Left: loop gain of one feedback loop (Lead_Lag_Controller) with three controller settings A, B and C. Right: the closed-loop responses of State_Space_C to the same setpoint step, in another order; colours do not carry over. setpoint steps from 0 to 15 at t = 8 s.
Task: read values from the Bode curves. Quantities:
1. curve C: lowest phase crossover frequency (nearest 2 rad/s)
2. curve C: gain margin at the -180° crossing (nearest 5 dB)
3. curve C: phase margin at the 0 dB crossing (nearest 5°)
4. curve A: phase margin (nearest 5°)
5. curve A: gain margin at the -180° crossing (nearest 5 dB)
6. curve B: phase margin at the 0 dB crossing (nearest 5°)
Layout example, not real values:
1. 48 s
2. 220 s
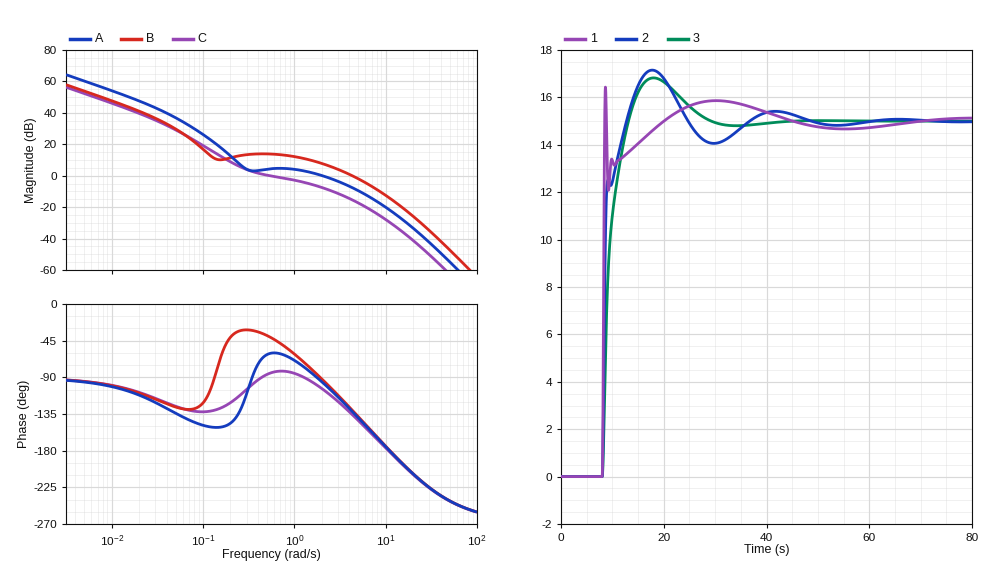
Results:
1. 10 rad/s
2. 30 dB
3. 95°
4. 85°
5. 20 dB
6. 50°
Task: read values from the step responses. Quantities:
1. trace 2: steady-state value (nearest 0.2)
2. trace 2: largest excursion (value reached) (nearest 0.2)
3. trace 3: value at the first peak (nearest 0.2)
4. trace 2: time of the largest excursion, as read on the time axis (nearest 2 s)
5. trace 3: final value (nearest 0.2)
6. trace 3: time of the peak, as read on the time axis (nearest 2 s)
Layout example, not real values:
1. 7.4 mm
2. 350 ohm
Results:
1. 15.0
2. 17.2
3. 16.8
4. 18 s
5. 15.0
6. 18 s
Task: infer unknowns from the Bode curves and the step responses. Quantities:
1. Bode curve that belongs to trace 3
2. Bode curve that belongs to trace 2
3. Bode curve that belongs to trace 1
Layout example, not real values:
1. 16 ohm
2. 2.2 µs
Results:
1. C
2. A
3. B
